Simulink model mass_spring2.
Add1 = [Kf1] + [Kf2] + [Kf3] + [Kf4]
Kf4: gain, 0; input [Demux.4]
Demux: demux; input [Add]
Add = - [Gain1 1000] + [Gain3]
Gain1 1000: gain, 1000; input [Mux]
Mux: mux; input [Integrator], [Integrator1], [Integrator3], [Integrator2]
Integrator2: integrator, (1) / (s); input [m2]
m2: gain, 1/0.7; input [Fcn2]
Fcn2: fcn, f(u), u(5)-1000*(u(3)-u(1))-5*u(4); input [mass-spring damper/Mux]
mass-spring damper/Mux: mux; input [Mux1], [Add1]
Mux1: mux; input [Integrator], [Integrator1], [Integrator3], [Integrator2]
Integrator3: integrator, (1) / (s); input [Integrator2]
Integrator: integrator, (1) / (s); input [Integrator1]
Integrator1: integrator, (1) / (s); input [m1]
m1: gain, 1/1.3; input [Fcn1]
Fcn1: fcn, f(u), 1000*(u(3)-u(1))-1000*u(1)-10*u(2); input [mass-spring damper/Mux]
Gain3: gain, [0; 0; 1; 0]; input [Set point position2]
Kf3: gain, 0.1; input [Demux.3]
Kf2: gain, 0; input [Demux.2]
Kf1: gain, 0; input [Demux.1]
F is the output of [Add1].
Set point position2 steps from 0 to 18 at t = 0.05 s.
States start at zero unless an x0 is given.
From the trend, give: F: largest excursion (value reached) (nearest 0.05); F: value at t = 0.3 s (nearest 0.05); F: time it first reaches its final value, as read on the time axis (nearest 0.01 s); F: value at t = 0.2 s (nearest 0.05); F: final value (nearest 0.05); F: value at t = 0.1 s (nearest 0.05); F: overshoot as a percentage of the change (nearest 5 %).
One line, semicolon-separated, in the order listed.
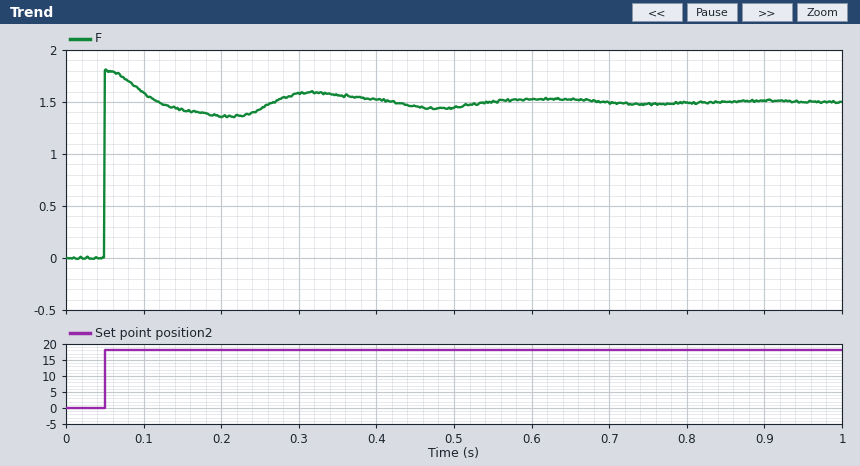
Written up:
1.80; 1.60; 0.05 s; 1.35; 1.50; 1.60; 20 %
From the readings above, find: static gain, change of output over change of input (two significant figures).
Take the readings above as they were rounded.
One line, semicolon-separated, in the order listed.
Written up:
0.083
